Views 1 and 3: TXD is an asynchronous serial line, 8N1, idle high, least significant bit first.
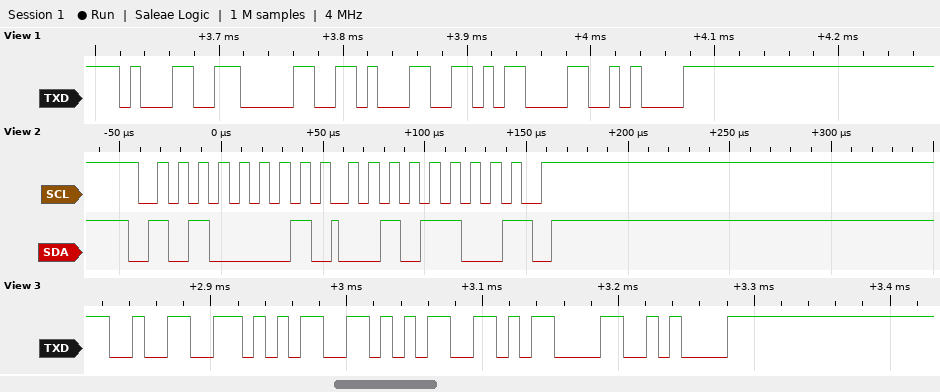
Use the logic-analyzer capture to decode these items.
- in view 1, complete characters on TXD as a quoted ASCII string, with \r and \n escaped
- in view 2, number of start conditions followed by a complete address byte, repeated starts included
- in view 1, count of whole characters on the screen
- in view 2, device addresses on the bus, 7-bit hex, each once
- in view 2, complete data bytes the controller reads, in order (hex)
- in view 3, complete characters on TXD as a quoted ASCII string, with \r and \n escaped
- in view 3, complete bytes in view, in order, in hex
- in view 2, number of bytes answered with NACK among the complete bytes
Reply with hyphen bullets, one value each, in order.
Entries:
- "101\r\n"
- 1
- 5
- 0x50
- 2C
- "255\r\n"
- 0x32 0x35 0x35 0x0D 0x0A
- 1
